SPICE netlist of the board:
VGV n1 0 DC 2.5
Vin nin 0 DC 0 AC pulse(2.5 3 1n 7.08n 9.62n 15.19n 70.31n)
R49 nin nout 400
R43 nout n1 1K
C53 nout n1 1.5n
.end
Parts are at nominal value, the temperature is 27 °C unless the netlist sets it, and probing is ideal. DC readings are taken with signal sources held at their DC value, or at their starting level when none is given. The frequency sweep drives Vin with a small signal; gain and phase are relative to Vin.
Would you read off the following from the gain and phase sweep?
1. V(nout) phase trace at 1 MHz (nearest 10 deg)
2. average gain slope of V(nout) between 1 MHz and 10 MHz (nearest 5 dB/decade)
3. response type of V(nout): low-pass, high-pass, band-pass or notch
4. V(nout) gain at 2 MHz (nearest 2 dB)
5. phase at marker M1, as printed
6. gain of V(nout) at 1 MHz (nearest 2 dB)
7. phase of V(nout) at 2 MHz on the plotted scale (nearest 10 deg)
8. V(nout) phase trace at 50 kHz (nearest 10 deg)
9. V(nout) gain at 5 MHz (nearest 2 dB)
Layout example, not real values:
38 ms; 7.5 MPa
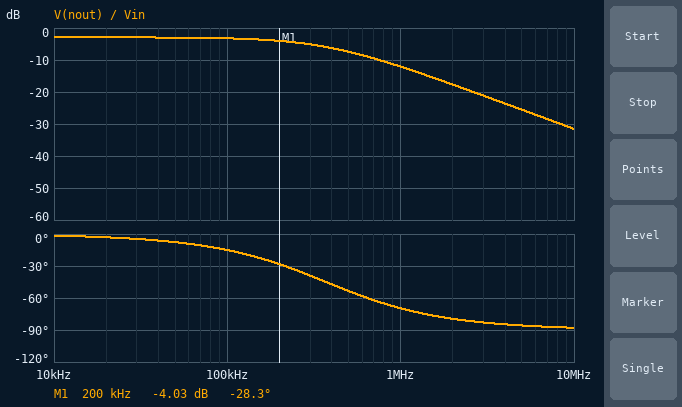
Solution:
-70 deg; -20 dB/decade; low-pass; -18 dB; -28.3 deg; -12 dB; -80 deg; -10 deg; -26 dB
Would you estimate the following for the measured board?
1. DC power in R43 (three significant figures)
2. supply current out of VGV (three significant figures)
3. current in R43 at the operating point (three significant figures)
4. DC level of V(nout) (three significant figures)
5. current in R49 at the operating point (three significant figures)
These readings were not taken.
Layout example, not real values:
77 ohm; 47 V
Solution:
3.19 mW; 1.79 mA; 1.79 mA; 714 mV; 1.79 mA
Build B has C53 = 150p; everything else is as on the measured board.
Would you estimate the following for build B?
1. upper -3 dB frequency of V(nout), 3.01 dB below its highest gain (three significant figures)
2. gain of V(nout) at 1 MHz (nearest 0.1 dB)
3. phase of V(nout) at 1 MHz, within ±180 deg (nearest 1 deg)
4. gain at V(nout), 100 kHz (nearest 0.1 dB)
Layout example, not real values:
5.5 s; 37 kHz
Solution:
3.71 MHz; -3.2 dB; -15 deg; -2.9 dB
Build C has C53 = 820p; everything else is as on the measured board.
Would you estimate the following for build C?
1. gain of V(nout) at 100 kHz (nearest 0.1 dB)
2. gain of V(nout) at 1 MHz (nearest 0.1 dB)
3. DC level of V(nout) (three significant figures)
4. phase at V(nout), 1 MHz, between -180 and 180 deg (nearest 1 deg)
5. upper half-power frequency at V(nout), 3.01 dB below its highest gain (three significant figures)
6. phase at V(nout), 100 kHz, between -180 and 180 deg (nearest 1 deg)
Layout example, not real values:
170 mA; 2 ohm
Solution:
-3.0 dB; -7.9 dB; 714 mV; -56 deg; 679 kHz; -8 deg
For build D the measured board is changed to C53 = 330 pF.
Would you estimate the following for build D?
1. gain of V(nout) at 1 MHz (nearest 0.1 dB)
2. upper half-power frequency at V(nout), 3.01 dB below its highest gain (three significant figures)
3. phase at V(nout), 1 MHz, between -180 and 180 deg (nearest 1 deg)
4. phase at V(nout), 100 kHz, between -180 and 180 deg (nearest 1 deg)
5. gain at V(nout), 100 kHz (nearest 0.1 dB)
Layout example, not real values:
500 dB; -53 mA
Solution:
-4.2 dB; 1.69 MHz; -31 deg; -3 deg; -2.9 dB
